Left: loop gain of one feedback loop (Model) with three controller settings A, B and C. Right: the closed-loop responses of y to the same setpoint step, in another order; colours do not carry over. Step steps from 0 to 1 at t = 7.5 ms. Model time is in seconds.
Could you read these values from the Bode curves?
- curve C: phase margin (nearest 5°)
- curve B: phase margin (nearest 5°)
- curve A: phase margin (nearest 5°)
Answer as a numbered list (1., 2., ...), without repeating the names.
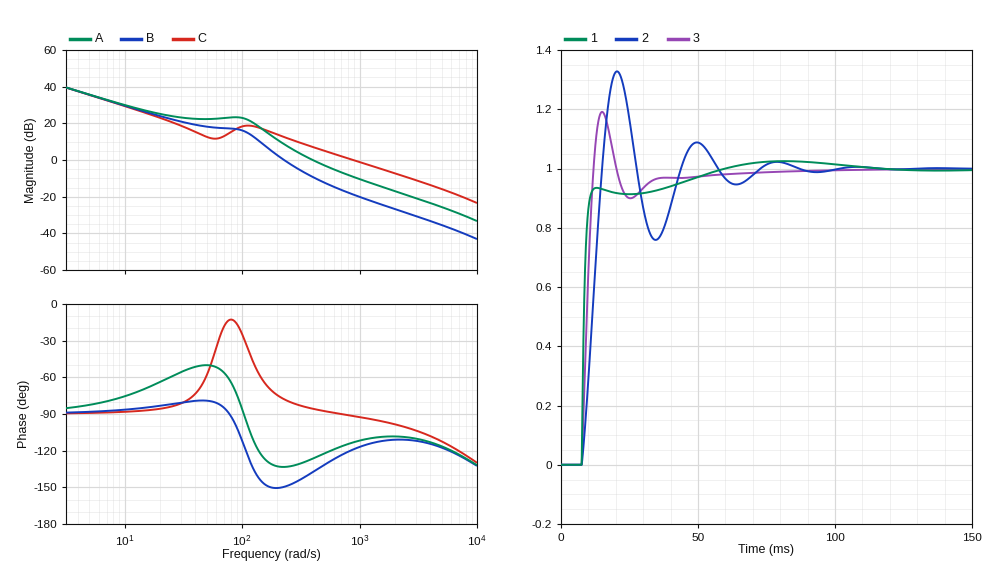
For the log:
1. 90°
2. 30°
3. 55°
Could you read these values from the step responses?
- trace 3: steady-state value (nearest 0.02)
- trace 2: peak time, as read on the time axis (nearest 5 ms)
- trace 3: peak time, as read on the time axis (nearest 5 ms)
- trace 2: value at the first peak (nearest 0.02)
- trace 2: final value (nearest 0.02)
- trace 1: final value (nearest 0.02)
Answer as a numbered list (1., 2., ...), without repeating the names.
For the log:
1. 1.00
2. 20 ms
3. 15 ms
4. 1.32
5. 1.00
6. 1.00
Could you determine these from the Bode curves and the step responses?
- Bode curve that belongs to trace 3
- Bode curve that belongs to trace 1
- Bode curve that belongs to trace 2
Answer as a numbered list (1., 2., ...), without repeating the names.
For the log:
1. A
2. C
3. B
